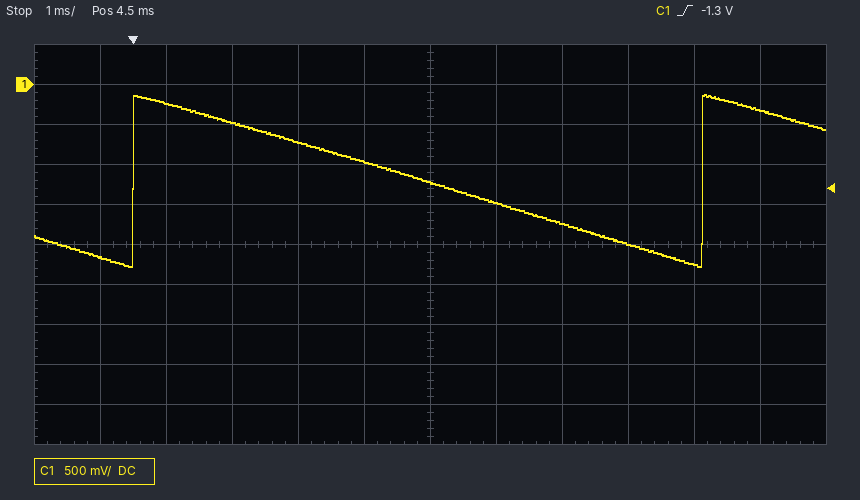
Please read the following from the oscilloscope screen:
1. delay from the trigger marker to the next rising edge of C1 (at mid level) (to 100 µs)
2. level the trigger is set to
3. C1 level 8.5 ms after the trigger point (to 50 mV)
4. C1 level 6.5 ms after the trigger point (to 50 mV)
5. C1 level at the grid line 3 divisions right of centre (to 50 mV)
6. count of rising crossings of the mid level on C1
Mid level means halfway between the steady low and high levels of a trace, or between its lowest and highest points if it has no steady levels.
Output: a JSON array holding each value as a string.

["8.6 ms", "-1.3 V", "-2.25 V", "-1.75 V", "-2.00 V", "2"]
